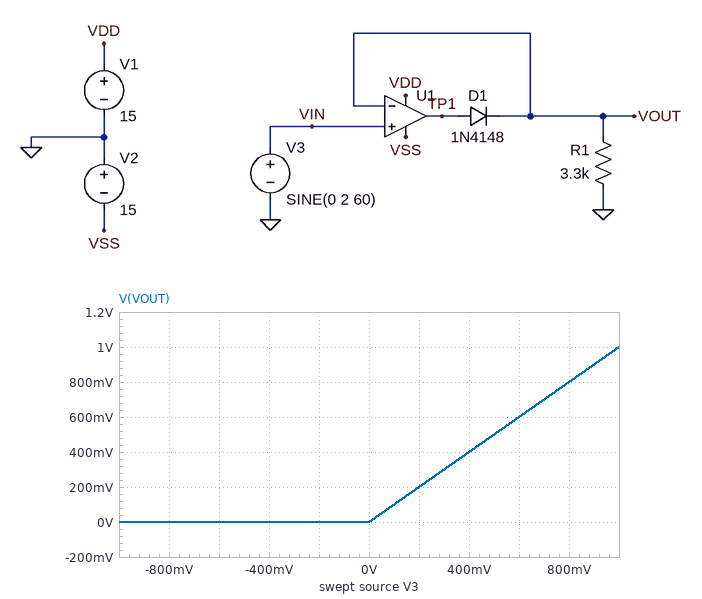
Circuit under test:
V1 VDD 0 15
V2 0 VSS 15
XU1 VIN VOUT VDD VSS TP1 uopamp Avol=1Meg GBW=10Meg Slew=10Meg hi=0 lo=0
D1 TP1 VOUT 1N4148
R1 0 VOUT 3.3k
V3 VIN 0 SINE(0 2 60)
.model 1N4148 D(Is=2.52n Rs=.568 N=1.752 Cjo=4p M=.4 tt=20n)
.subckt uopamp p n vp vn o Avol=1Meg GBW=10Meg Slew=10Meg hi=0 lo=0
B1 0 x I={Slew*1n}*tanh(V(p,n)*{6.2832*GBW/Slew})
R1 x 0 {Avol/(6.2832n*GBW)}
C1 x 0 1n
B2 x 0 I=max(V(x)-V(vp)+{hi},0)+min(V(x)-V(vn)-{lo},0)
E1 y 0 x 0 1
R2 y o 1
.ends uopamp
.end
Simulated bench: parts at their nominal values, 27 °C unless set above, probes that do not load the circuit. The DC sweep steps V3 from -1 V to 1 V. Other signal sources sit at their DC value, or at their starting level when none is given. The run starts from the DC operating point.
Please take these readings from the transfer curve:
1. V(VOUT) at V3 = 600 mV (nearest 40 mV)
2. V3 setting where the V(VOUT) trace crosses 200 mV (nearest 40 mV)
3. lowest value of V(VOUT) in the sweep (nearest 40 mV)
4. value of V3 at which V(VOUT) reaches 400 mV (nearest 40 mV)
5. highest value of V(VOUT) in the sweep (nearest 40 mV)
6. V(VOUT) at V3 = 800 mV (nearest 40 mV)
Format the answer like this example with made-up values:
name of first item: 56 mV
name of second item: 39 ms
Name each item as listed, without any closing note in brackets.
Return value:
V(VOUT) at V3 = 600 mV: 600 mV
V3 setting where the V(VOUT) trace crosses 200 mV: 200 mV
lowest value of V(VOUT) in the sweep: 0 V
value of V3 at which V(VOUT) reaches 400 mV: 400 mV
highest value of V(VOUT) in the sweep: 1.00 V
V(VOUT) at V3 = 800 mV: 800 mV
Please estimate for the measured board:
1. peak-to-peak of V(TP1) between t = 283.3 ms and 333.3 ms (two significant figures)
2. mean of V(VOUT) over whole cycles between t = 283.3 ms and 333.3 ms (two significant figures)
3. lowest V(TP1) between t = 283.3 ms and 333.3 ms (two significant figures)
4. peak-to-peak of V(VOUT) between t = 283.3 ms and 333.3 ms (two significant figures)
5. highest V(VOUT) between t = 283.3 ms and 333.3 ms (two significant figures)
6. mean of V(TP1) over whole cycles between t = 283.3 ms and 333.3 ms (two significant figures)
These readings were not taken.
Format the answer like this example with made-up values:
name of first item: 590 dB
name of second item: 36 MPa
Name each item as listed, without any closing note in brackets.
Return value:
peak-to-peak of V(TP1) between t = 283.3 ms and 333.3 ms: 18 V
mean of V(VOUT) over whole cycles between t = 283.3 ms and 333.3 ms: 640 mV
lowest V(TP1) between t = 283.3 ms and 333.3 ms: -15 V
peak-to-peak of V(VOUT) between t = 283.3 ms and 333.3 ms: 2.0 V
highest V(VOUT) between t = 283.3 ms and 333.3 ms: 2.0 V
mean of V(TP1) over whole cycles between t = 283.3 ms and 333.3 ms: -6.6 V
